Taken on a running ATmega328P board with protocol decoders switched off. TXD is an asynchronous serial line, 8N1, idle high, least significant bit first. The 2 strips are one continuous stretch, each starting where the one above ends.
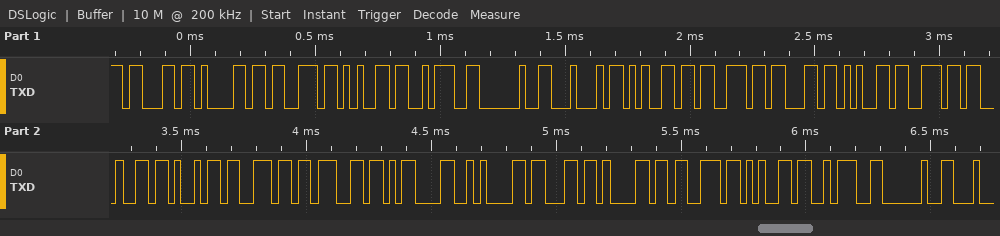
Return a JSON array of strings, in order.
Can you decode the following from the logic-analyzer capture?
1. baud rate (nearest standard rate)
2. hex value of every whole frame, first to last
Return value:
["38400 baud", "0x63 0x61 0x73 0x65 0x3A 0x20 0x44 0x65 0x73 0x63 0x65 0x6E 0x64 0x69 0x6E 0x67 0x0D 0x0A 0x63 0x61 0x73 0x65 0x3A 0x20"]
